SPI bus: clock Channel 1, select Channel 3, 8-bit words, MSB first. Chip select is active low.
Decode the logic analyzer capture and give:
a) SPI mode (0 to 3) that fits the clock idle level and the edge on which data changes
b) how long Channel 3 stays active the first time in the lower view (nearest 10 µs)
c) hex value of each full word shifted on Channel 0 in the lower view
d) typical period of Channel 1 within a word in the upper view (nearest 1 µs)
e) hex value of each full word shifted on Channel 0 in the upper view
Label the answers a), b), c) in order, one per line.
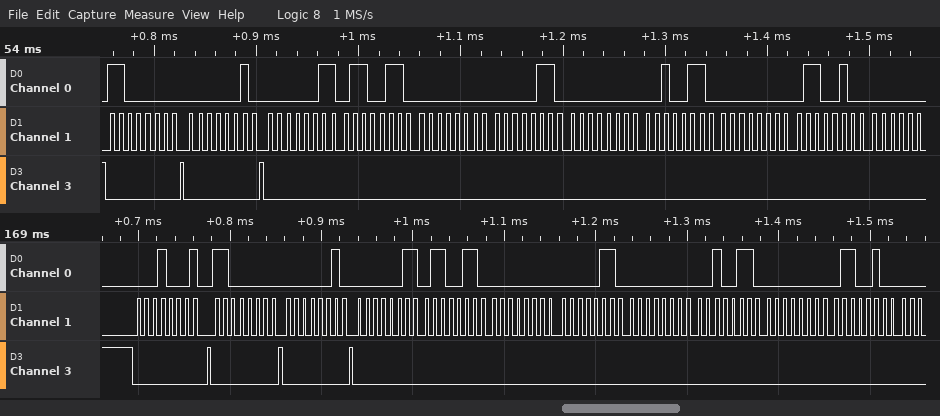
a) 0
b) 80 µs
c) 11, C0, 02, 03, 66, 00, 06, 00, 26, 00, 64
d) 9 µs
e) C0, 02, 03, 66, 00, 06, 00, 26, 00, 64
